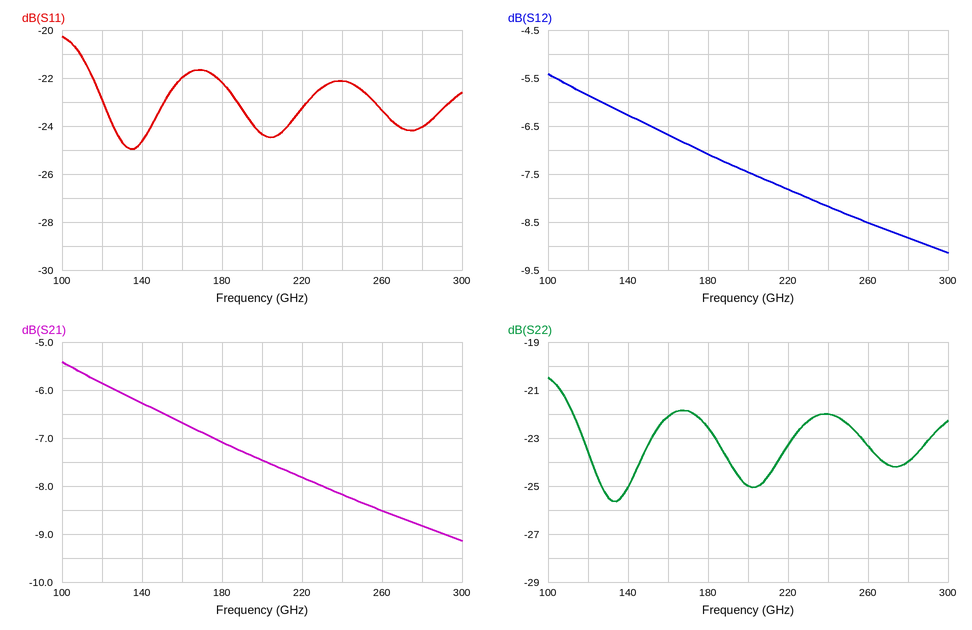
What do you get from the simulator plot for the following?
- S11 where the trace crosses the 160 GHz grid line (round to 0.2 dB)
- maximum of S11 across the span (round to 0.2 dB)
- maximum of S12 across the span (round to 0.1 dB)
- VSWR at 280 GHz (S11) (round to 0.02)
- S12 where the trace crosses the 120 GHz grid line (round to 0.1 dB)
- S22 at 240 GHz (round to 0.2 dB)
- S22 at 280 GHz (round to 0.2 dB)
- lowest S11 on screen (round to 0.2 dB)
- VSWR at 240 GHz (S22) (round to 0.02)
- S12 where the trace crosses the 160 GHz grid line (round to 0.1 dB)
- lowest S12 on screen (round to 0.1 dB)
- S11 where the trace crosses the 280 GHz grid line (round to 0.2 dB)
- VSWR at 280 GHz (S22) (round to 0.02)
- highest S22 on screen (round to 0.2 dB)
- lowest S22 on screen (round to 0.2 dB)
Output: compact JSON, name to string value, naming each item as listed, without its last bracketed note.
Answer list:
{"S11 where the trace crosses the 160 GHz grid line": "-22.0 dB", "maximum of S11 across the span": "-20.2 dB", "maximum of S12 across the span": "-5.4 dB", "VSWR at 280 GHz (S11)": "1.14", "S12 where the trace crosses the 120 GHz grid line": "-5.9 dB", "S22 at 240 GHz": "-22.0 dB", "S22 at 280 GHz": "-24.0 dB", "lowest S11 on screen": "-25.0 dB", "VSWR at 240 GHz (S22)": "1.18", "S12 where the trace crosses the 160 GHz grid line": "-6.7 dB", "lowest S12 on screen": "-9.1 dB", "S11 where the trace crosses the 280 GHz grid line": "-24.0 dB", "VSWR at 280 GHz (S22)": "1.14", "highest S22 on screen": "-20.4 dB", "lowest S22 on screen": "-25.6 dB"}
